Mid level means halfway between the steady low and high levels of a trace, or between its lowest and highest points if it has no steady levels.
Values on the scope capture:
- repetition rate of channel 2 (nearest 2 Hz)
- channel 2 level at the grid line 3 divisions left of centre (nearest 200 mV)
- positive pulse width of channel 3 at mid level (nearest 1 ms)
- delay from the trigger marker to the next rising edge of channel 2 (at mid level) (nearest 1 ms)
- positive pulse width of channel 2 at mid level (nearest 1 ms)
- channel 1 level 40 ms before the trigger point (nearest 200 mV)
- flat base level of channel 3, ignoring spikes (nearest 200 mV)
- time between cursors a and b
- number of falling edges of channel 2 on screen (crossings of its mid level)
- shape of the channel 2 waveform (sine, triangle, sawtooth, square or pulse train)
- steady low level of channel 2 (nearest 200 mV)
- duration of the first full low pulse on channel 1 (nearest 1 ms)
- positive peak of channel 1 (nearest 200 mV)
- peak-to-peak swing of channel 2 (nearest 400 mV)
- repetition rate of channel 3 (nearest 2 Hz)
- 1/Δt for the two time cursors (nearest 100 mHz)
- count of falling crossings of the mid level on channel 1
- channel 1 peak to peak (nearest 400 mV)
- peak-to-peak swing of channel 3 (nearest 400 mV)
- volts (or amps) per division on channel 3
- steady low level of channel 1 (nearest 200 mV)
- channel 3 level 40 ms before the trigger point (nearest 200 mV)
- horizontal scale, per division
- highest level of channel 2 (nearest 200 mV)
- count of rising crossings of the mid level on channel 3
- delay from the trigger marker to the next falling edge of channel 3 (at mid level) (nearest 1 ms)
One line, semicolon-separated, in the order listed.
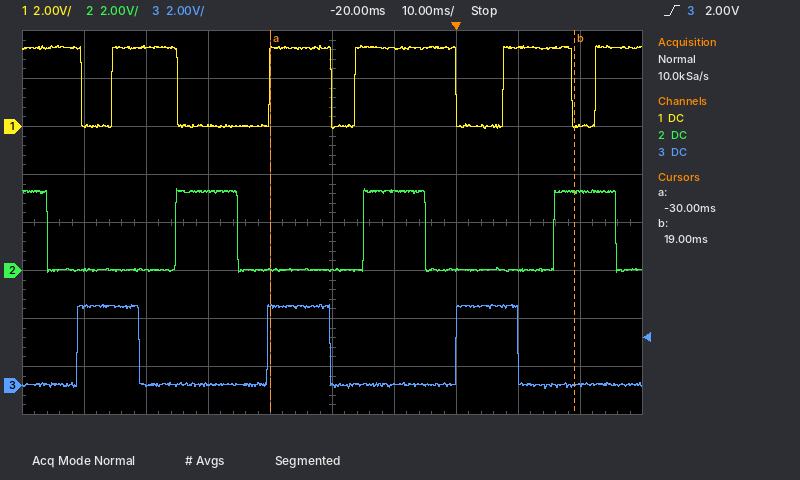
32 Hz; 0.0 V; 10 ms; 16 ms; 10 ms; 0.0 V; 0.0 V; 49 ms; 4; pulse train; 0.0 V; 5 ms; 3.4 V; 3.6 V; 32 Hz; 20.4 Hz; 5; 3.6 V; 3.6 V; 2 V; 0.0 V; 0.0 V; 10 ms; 3.4 V; 3; 10 ms
